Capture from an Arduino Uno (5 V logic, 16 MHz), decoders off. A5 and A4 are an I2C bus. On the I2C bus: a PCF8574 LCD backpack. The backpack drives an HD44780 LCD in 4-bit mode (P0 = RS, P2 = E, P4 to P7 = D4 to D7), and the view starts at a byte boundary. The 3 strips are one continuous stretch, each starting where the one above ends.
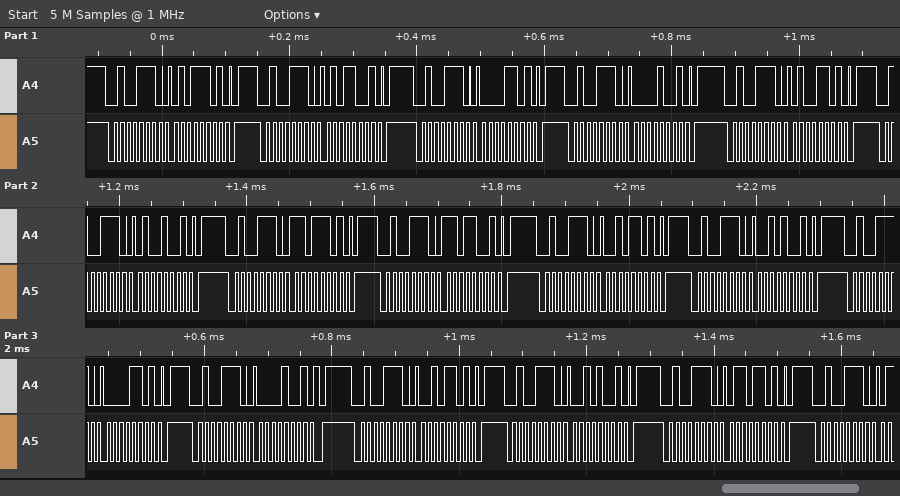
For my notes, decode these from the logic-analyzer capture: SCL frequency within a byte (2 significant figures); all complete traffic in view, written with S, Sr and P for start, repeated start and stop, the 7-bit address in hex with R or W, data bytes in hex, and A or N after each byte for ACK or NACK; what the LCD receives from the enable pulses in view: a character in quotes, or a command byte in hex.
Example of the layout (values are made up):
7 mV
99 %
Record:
100 kHz
S 27W A 5D A P S 27W A 59 A P S 27W A 0D A P S 27W A 09 A P S 27W A 4D A P S 27W A 49 A P S 27W A DD A P S 27W A D9 A P S 27W A 2D A P S 27W A 29 A P S 27W A 0D A P S 27W A 09 A P S 27W A 2D A P S 27W A 29 A P S 27W A 6D A P S 27W A
'P' 'M' ' '
